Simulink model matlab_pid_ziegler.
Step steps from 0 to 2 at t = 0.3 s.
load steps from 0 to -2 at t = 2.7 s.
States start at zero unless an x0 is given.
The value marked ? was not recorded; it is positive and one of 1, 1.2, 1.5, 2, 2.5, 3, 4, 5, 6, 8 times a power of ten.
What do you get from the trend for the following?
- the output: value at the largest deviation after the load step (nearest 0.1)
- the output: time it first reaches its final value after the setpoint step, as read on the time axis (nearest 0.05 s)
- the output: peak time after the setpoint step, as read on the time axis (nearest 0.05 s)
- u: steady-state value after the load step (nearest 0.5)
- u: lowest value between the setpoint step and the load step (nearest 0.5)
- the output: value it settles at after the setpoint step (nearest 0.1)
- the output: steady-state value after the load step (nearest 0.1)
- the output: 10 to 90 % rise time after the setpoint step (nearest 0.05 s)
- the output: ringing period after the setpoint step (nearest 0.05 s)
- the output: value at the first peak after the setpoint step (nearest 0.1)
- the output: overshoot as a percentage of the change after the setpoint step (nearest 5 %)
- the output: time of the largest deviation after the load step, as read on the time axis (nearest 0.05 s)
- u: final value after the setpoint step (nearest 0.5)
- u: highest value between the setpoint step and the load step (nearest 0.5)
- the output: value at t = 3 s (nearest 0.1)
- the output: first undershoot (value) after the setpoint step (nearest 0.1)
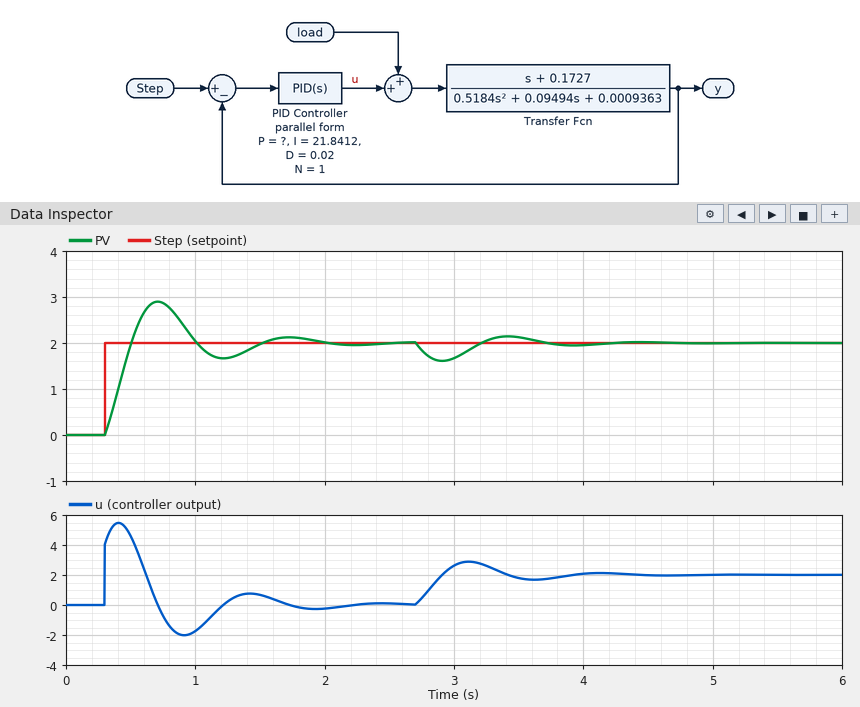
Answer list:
1.6
0.50 s
0.70 s
2.0
-2.0
2.0
2.0
0.15 s
1.00 s
2.9
45 %
2.90 s
0.0
5.5
1.7
1.7
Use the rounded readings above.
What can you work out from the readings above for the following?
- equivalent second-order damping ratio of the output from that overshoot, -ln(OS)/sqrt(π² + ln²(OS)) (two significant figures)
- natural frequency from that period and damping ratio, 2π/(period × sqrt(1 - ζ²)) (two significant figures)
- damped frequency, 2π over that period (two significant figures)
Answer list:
0.25
6.5 rad/s
6.3 rad/s
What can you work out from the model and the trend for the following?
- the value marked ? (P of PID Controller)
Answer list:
2
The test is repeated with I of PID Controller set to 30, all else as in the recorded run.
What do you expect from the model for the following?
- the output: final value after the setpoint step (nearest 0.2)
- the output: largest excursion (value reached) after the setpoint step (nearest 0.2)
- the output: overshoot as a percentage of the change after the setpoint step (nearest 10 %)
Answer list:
2.0
3.0
50 %
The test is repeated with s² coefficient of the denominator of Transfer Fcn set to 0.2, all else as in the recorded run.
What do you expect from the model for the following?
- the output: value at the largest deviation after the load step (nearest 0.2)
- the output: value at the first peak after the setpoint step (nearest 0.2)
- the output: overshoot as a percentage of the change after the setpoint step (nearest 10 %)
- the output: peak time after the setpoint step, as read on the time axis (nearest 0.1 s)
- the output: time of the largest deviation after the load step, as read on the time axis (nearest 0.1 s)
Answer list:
1.4
2.6
30 %
0.5 s
2.8 s
